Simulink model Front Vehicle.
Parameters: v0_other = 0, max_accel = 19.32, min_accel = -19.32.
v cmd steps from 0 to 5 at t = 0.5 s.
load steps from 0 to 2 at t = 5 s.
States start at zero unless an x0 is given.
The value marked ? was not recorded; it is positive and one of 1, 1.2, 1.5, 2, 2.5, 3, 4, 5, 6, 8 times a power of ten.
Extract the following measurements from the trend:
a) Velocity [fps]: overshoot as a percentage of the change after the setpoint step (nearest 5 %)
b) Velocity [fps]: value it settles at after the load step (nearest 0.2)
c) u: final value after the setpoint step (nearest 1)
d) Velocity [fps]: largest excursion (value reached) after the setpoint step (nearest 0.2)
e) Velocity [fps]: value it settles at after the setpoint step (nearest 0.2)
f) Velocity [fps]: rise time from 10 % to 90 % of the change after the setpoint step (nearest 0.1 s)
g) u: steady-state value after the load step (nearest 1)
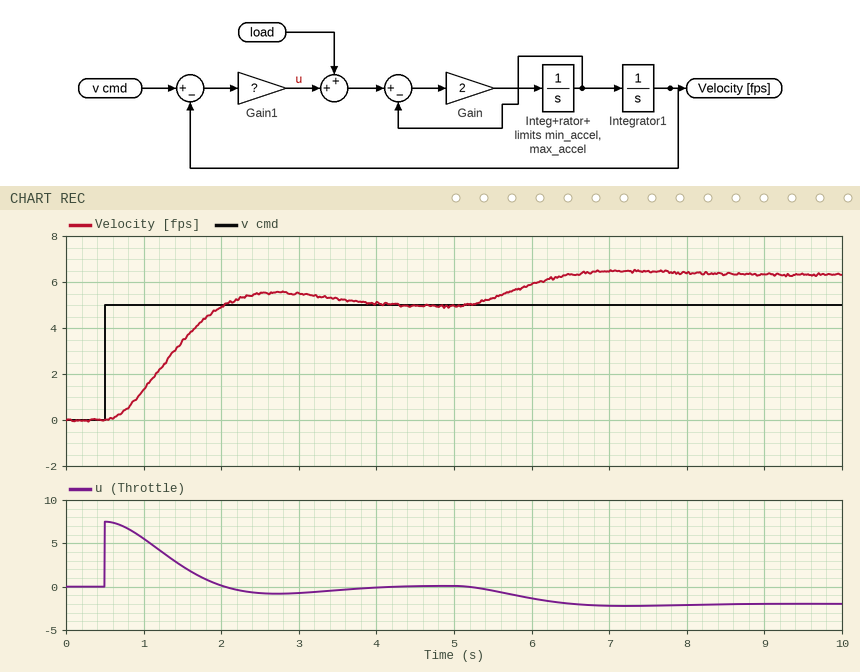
10 %
6.4
0
5.6
5.0
1.0 s
-2
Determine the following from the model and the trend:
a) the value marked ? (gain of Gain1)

1.5
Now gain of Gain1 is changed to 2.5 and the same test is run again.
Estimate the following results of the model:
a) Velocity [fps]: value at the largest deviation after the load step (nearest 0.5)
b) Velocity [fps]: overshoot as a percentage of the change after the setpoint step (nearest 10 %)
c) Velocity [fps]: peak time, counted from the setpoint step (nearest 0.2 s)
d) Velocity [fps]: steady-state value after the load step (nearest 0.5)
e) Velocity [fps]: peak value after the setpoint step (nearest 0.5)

6.0
20 %
1.6 s
6.0
6.0
